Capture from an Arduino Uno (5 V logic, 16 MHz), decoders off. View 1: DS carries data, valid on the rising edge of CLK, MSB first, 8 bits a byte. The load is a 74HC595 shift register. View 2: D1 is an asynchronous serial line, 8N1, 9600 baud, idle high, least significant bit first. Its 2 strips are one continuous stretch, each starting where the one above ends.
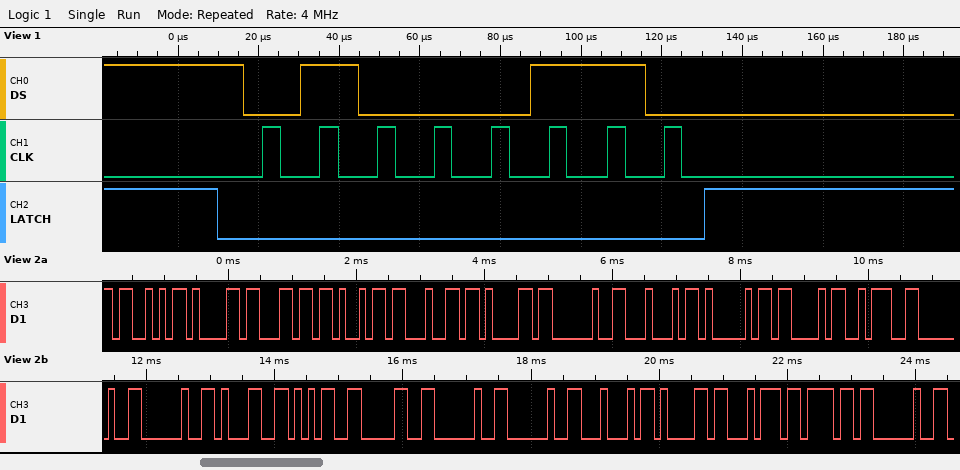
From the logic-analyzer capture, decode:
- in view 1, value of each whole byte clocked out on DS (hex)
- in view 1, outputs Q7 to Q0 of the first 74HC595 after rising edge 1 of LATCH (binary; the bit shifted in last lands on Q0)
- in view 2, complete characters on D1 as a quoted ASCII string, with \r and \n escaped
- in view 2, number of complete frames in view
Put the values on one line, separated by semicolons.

46; 01000110; "Salida DAC:  150  Dato "; 23
